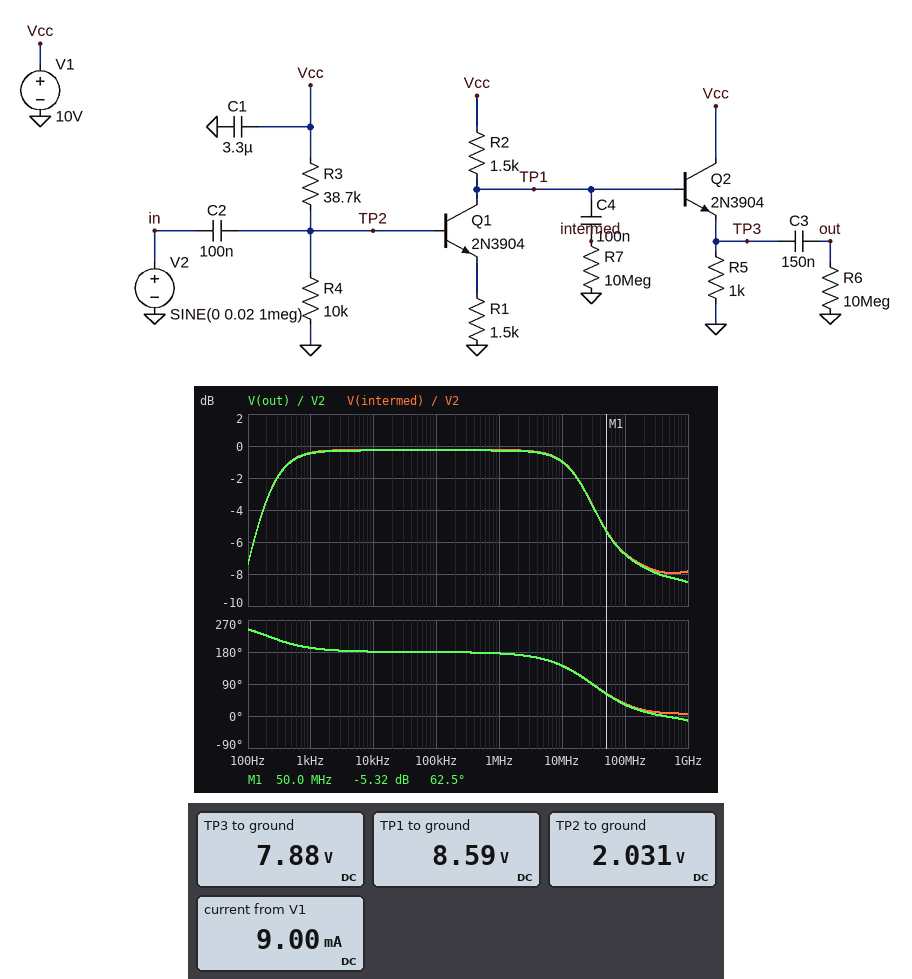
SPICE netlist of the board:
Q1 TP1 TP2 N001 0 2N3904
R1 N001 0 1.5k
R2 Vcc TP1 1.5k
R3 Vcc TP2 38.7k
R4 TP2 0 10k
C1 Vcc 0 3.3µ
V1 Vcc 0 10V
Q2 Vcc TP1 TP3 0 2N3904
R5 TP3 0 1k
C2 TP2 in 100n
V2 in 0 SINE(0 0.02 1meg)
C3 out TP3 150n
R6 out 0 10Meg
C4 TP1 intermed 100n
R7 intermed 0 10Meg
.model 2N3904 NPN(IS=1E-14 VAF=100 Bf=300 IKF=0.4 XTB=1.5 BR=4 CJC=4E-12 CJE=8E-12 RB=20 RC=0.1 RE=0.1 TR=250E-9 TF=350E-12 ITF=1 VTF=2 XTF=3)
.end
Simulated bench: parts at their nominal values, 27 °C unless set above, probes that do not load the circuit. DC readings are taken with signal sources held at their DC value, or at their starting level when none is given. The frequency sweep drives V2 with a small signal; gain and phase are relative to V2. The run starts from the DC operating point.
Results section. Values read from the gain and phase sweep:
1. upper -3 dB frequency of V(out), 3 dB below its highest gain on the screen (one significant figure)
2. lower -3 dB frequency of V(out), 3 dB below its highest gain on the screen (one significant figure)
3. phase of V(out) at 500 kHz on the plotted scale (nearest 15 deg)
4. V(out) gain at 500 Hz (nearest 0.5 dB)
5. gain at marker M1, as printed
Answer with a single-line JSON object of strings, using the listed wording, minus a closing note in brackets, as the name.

{"upper -3 dB frequency of V(out), 3 dB below its highest gain on the screen": "30 MHz", "lower -3 dB frequency of V(out), 3 dB below its highest gain on the screen": "200 Hz", "phase of V(out) at 500 kHz on the plotted scale": "180 deg", "V(out) gain at 500 Hz": "-1.0 dB", "gain at marker M1, as printed": "-5.32 dB"}
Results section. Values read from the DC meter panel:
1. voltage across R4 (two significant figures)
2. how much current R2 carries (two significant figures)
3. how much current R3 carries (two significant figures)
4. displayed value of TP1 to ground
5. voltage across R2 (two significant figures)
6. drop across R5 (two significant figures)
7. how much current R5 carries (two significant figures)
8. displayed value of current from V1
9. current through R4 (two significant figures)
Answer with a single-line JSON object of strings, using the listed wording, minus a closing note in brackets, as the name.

{"voltage across R4": "2.0 V", "how much current R2 carries": "940 µA", "how much current R3 carries": "210 µA", "displayed value of TP1 to ground": "8.59 V", "voltage across R2": "1.4 V", "drop across R5": "7.9 V", "how much current R5 carries": "7.9 mA", "displayed value of current from V1": "9.00 mA", "current through R4": "200 µA"}
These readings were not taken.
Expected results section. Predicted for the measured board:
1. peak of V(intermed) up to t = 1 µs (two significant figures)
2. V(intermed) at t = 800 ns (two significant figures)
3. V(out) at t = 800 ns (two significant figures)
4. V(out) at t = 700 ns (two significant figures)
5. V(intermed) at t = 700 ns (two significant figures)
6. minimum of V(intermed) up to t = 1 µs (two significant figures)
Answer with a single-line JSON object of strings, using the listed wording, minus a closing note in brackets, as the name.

{"peak of V(intermed) up to t = 1 µs": "19 mV", "V(intermed) at t = 800 ns": "19 mV", "V(out) at t = 800 ns": "19 mV", "V(out) at t = 700 ns": "18 mV", "V(intermed) at t = 700 ns": "18 mV", "minimum of V(intermed) up to t = 1 µs": "-19 mV"}
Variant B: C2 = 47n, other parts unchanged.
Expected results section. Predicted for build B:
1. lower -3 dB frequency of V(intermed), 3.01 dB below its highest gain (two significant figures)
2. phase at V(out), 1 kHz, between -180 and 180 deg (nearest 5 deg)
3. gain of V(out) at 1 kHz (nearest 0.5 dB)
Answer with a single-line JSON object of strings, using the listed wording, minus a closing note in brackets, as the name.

{"lower -3 dB frequency of V(intermed), 3.01 dB below its highest gain": "430 Hz", "phase at V(out), 1 kHz, between -180 and 180 deg": "-155 deg", "gain of V(out) at 1 kHz": "-1.0 dB"}
